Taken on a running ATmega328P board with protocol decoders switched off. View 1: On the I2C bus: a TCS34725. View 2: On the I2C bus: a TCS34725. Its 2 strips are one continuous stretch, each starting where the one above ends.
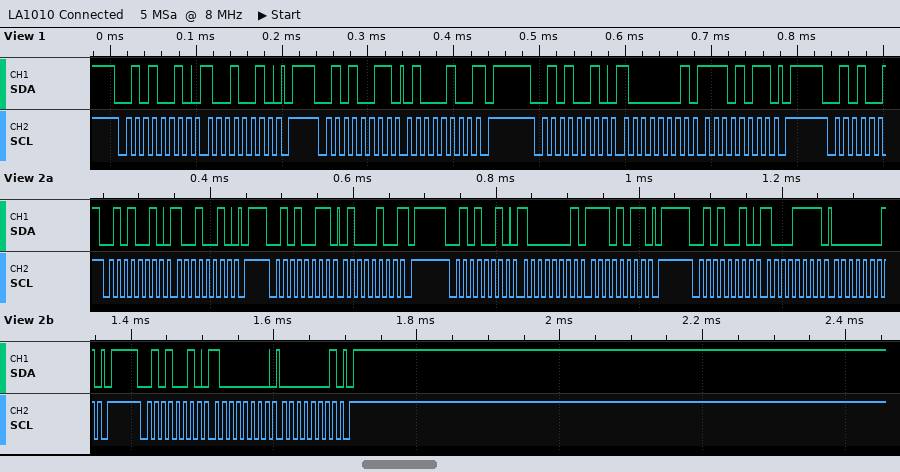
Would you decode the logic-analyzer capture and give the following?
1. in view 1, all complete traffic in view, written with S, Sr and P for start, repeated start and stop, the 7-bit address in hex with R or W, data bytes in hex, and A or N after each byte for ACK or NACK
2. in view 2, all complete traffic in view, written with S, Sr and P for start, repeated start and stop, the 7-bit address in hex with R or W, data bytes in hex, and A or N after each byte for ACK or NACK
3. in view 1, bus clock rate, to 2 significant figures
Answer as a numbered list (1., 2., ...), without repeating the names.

1. S 29W A 92 A P S 29R A 44 N P S 29W A 81 A EB A P
2. S 29W A 92 A P S 29R A 44 N P S 29W A 81 A EB A P S 29W A 8F A 01 A P S 29W A 80 A 01 A P
3. 100 kHz
